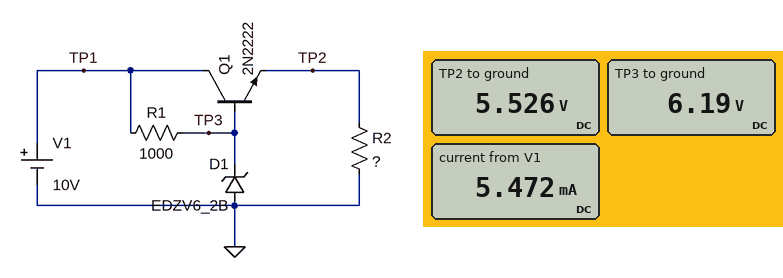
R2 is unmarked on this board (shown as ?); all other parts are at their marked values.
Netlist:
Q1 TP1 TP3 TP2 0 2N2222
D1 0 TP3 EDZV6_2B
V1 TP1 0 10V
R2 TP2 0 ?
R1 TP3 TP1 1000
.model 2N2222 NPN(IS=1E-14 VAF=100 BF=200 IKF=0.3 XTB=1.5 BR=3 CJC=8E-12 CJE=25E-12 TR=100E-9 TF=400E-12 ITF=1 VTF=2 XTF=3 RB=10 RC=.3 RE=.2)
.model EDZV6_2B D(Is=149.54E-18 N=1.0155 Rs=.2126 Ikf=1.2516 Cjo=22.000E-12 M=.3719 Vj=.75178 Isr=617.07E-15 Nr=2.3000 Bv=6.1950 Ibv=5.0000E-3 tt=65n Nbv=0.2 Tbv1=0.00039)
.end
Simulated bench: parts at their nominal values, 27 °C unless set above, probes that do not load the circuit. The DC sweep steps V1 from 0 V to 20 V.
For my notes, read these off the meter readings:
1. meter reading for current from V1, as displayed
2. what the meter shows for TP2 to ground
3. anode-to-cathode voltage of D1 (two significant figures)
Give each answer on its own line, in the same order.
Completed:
5.472 mA
5.526 V
-6.2 V
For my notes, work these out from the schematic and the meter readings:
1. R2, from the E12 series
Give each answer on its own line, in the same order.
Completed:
3.3 kΩ
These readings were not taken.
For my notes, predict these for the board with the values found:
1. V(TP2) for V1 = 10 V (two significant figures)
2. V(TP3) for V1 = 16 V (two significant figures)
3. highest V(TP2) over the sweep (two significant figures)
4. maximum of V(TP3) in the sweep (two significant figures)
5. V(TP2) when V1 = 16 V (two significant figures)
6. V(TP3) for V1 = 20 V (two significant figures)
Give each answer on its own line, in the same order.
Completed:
5.5 V
6.2 V
5.5 V
6.2 V
5.5 V
6.2 V
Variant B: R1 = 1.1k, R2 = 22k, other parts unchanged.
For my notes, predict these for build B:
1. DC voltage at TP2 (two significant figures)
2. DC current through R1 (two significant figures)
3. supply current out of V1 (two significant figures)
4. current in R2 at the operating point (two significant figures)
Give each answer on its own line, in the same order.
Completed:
5.6 V
3.5 mA
3.7 mA
250 µA
